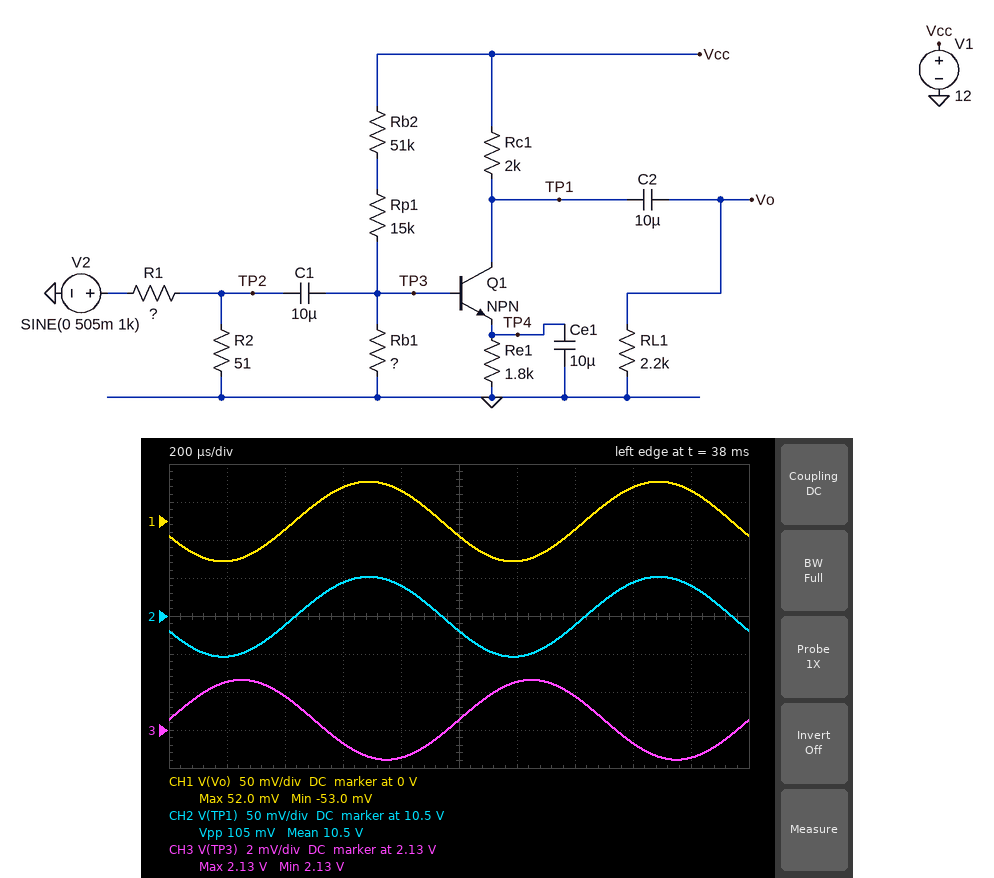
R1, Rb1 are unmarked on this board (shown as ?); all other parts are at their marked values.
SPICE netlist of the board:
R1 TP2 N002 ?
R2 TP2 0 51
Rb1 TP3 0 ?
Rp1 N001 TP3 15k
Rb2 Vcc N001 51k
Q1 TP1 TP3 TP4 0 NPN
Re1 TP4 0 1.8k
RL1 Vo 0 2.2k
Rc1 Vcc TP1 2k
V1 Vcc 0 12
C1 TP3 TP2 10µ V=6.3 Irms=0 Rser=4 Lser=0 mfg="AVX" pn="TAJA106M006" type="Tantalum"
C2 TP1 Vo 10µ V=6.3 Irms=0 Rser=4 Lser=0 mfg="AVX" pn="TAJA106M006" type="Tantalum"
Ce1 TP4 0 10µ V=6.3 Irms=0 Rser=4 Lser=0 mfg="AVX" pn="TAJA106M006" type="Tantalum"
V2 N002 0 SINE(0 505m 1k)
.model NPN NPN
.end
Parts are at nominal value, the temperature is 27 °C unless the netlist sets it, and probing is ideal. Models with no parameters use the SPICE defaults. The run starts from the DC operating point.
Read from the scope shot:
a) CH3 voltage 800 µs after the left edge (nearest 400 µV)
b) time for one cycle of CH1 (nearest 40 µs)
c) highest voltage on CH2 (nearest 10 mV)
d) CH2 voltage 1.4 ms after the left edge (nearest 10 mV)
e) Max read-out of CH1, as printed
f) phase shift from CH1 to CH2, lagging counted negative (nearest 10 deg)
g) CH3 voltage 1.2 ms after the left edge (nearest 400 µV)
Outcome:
2.1284 V
1.00 ms
10.55 V
10.49 V
52.0 mV
0 deg
2.1324 V
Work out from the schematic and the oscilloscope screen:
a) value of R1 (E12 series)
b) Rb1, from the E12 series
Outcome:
12 kΩ
15 kΩ
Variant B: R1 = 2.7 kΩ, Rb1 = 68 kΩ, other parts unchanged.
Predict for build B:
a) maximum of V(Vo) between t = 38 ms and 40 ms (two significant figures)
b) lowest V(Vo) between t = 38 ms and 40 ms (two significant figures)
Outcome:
430 mV
-450 mV
